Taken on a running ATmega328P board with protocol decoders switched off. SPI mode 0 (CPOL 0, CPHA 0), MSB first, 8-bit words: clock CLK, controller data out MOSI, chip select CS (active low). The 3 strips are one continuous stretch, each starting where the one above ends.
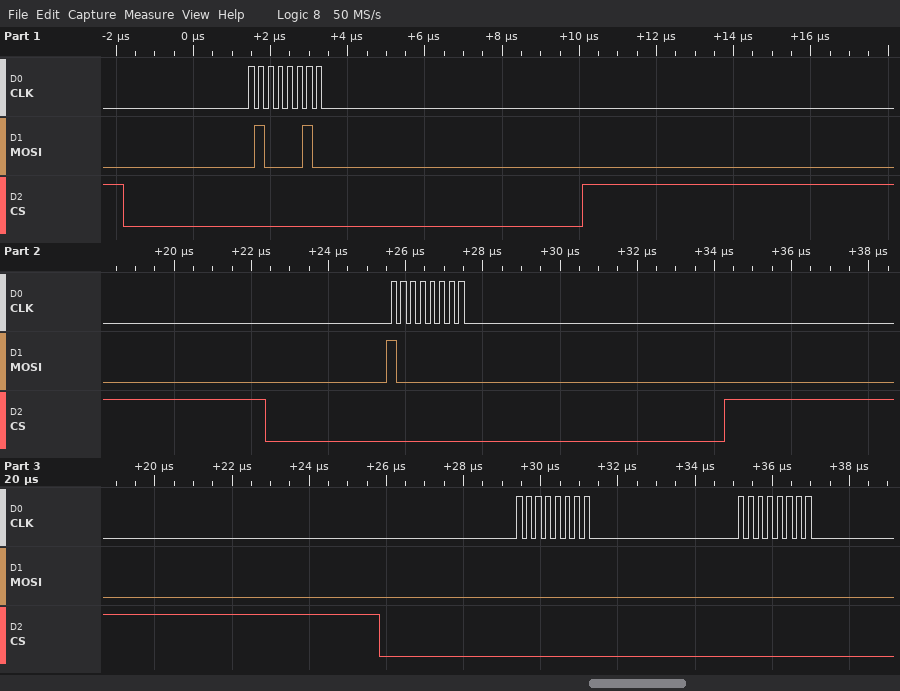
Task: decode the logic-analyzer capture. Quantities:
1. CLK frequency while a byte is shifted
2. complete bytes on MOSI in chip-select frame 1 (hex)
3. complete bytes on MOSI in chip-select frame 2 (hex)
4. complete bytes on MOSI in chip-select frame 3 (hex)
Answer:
4 MHz
42
80
00 00
